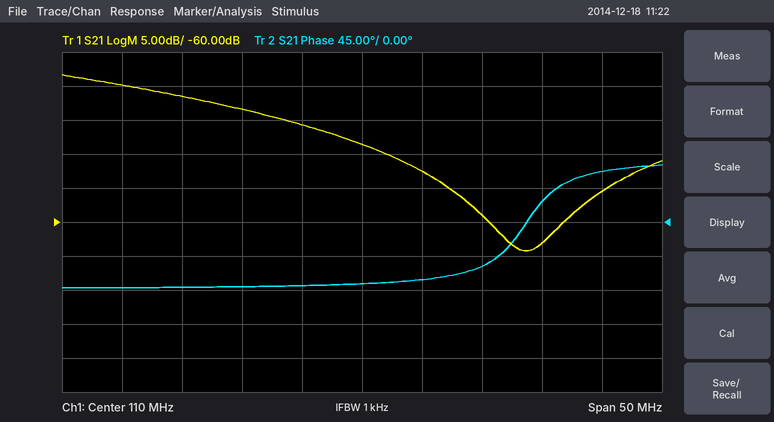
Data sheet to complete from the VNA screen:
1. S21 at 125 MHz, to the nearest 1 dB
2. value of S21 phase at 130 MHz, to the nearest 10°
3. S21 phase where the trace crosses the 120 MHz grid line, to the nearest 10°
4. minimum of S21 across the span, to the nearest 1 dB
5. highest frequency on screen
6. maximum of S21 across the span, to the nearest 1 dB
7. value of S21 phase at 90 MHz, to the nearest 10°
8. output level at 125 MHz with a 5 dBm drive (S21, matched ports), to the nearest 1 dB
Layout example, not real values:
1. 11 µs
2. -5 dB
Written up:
1. -63 dB
2. 70°
3. -60°
4. -64 dB
5. 135 MHz
6. -38 dB
7. -90°
8. -58 dBm
